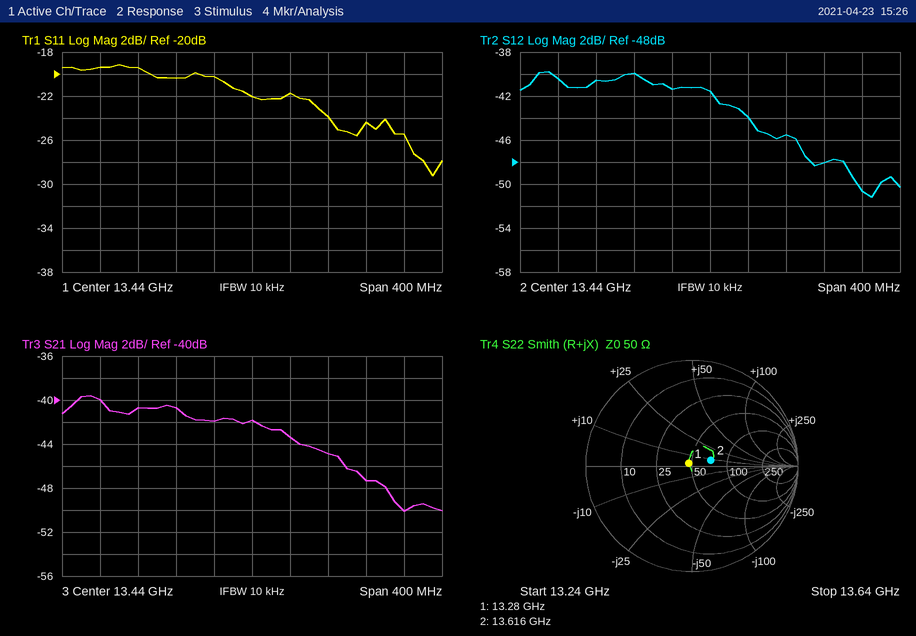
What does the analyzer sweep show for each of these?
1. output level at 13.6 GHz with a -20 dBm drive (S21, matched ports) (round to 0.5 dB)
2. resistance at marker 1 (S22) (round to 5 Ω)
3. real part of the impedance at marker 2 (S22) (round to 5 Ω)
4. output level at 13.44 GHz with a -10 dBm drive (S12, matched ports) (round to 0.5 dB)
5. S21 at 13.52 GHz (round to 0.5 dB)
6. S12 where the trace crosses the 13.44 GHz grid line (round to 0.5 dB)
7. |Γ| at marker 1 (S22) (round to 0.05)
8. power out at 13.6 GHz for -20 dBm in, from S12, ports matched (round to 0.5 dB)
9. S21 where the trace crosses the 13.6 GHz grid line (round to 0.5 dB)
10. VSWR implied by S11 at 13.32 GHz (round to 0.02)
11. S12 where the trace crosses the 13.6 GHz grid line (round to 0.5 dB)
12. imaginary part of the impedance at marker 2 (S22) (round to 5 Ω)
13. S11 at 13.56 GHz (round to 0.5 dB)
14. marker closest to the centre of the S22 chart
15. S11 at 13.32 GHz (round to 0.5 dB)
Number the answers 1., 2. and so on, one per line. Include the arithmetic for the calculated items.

1. -20 dBm + (-50.0 dB) = -70.0 dBm
2. 45 Ω
3. 70 Ω
4. -10 dBm + (-41.5 dB) = -51.5 dBm
5. -45.0 dB
6. -41.5 dB
7. 0.05
8. -20 dBm + (-50.5 dB) = -70.5 dBm
9. -50.0 dB
10. |Γ| = 10^(-19.5/20) = 0.1059; VSWR = (1 + 0.1059)/(1 − 0.1059) ≈ 1.24
11. -50.5 dB
12. +10 Ω
13. -24.5 dB
14. marker 1
15. -19.5 dB
